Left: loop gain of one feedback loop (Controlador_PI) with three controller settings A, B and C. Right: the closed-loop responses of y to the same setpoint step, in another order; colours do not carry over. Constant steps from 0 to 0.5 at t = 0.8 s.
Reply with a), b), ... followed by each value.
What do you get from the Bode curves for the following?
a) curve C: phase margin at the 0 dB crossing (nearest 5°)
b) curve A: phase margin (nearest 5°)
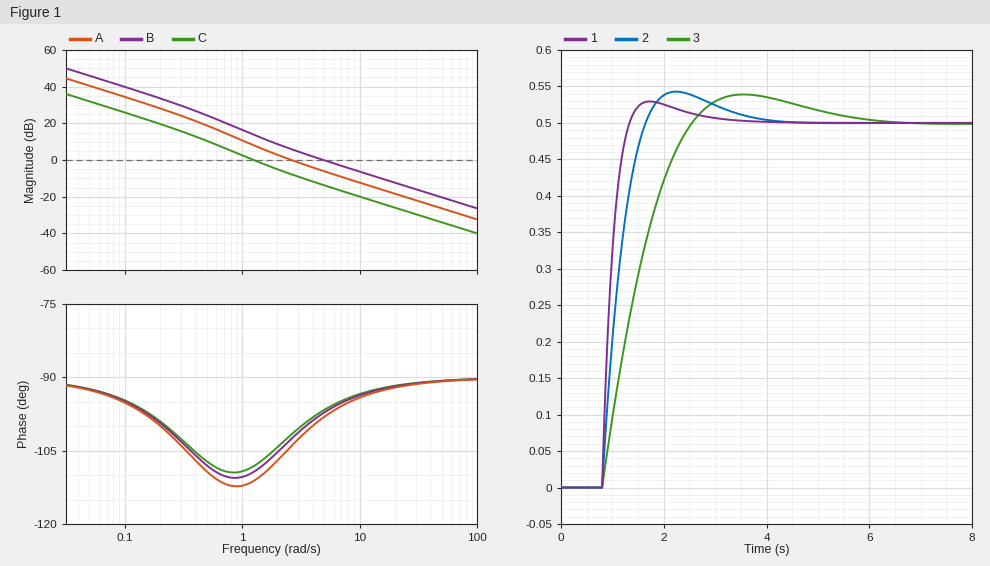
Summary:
a) 70°
b) 75°
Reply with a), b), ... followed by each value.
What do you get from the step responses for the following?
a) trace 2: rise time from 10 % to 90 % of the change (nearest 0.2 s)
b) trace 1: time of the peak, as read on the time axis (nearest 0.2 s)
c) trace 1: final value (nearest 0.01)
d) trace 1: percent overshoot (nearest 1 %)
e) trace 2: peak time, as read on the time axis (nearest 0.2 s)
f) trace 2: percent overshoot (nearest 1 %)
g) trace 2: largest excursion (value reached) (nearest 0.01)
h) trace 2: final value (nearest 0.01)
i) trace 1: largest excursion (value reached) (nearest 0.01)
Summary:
a) 0.6 s
b) 1.8 s
c) 0.50
d) 6 %
e) 2.2 s
f) 9 %
g) 0.54
h) 0.50
i) 0.53
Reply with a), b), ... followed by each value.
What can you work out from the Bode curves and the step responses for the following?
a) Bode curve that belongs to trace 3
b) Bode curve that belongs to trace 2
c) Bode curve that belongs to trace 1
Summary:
a) C
b) A
c) B
